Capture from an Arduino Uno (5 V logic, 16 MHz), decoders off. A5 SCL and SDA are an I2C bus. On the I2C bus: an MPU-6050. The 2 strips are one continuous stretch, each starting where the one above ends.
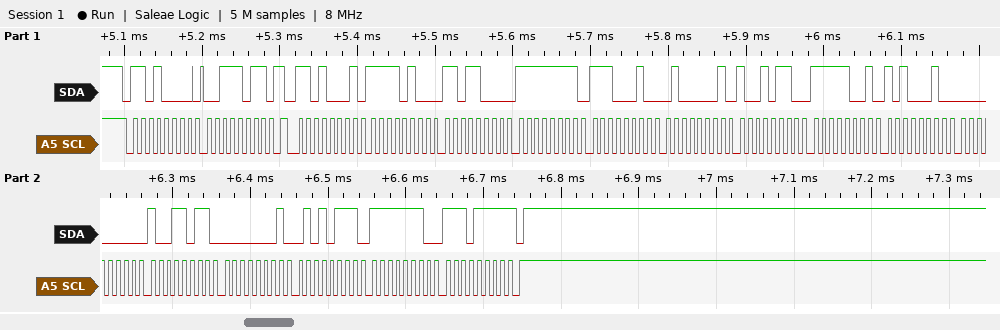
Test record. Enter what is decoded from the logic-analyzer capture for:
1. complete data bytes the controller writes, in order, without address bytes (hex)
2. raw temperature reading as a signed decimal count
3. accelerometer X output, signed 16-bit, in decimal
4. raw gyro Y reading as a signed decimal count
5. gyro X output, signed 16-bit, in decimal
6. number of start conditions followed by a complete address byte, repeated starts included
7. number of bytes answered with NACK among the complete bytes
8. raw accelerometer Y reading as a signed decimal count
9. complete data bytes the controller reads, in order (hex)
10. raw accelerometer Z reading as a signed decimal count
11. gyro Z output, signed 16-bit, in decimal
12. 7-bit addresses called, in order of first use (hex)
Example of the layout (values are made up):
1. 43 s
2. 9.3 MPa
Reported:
1. 3B
2. -1630
3. -2856
4. 343
5. 155
6. 2
7. 1
8. -30
9. F4 D8 FF E2 41 96 F9 A2 00 9B 01 57 FE EF
10. 16790
11. -273
12. 0x68
